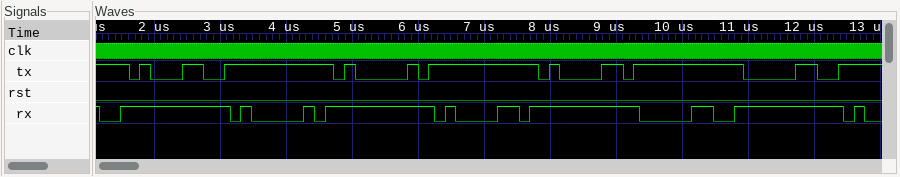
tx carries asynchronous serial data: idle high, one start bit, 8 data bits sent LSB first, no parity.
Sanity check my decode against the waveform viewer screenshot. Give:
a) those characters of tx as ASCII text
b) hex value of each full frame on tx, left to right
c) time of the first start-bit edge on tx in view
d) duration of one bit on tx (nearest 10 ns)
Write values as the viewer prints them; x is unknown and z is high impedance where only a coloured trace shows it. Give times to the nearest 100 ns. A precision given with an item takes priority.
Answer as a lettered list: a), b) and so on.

a) "1Aa0"
b) 31, 41, 61, 30
c) 1600 ns
d) 160 ns
